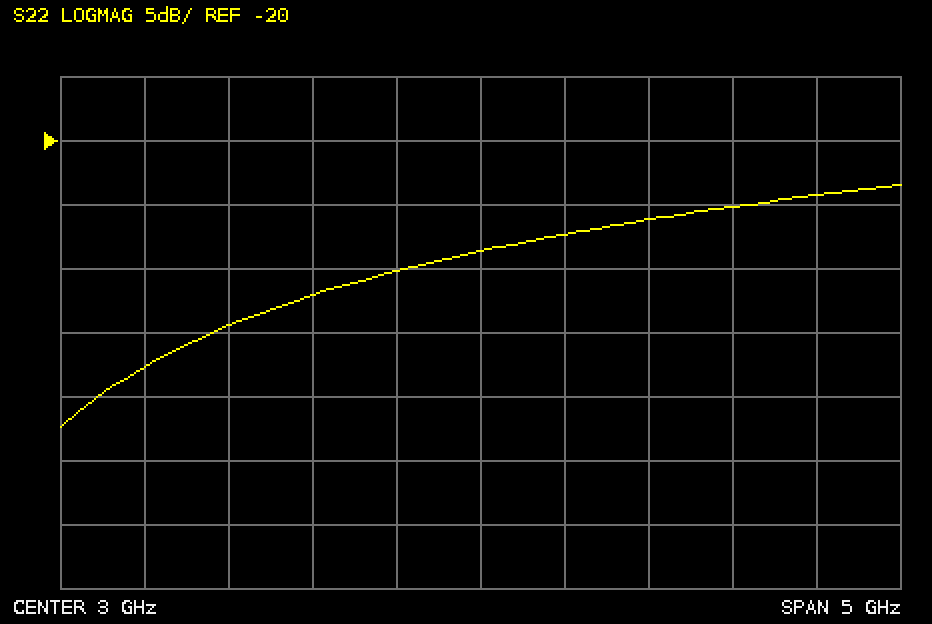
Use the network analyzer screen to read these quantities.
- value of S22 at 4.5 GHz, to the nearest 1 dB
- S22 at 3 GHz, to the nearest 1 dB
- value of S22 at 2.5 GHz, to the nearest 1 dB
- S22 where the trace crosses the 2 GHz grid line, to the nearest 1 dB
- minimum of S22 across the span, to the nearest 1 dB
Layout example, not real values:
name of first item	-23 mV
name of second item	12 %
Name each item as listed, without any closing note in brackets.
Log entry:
value of S22 at 4.5 GHz, to the nearest 1 dB	-25 dB
S22 at 3 GHz, to the nearest 1 dB	-29 dB
value of S22 at 2.5 GHz, to the nearest 1 dB	-30 dB
S22 where the trace crosses the 2 GHz grid line, to the nearest 1 dB	-32 dB
minimum of S22 across the span, to the nearest 1 dB	-42 dB
